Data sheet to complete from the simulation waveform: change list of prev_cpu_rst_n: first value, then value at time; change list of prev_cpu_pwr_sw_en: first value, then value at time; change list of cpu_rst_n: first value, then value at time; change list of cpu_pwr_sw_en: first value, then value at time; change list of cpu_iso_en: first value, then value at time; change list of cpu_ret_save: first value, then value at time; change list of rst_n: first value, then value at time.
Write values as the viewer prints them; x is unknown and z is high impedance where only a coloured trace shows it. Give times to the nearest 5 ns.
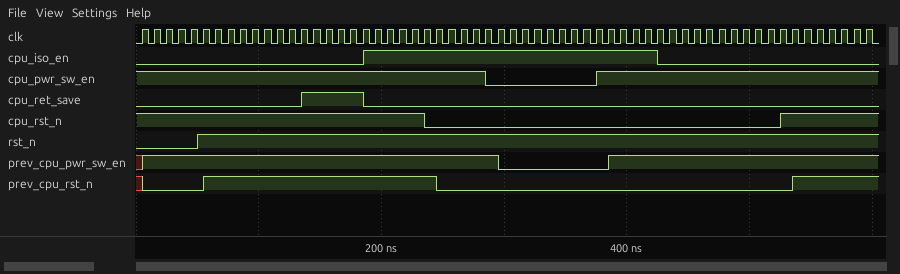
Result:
x, 0 at 5 ns, 1 at 55 ns, 0 at 245 ns, 1 at 535 ns
x, 1 at 5 ns, 0 at 295 ns, 1 at 385 ns
1, 0 at 235 ns, 1 at 525 ns
1, 0 at 285 ns, 1 at 375 ns
0, 1 at 185 ns, 0 at 425 ns
0, 1 at 135 ns, 0 at 185 ns
0, 1 at 50 ns
